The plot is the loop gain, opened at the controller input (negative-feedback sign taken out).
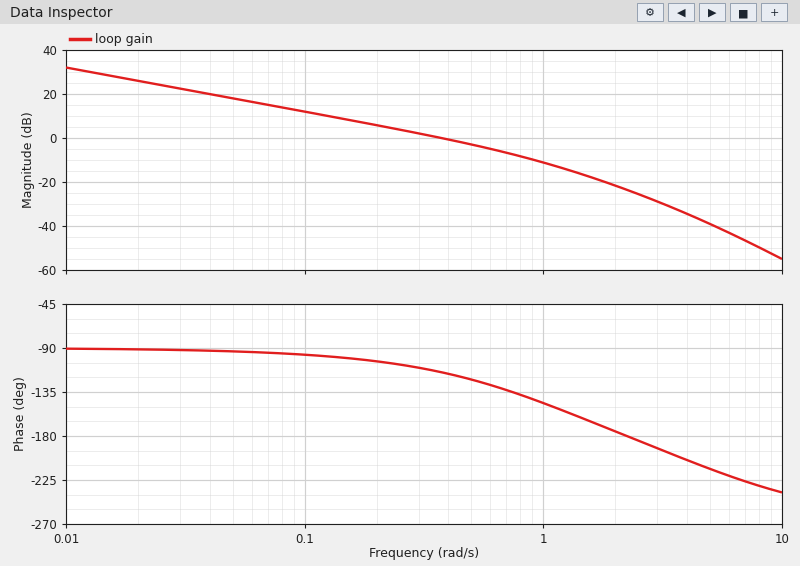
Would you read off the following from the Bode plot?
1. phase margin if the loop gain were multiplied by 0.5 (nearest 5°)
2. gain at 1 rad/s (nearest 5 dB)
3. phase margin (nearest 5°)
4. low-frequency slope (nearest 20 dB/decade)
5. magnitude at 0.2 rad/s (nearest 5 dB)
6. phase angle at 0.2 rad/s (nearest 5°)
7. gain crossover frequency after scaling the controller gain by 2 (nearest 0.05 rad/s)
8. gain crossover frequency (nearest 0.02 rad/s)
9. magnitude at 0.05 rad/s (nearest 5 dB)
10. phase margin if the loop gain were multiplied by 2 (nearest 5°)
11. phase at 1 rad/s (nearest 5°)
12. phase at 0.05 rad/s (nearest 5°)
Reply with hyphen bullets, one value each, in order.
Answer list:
- 75°
- -10 dB
- 65°
- -20 dB/decade
- 5 dB
- -105°
- 0.65 rad/s
- 0.38 rad/s
- 20 dB
- 50°
- -145°
- -95°
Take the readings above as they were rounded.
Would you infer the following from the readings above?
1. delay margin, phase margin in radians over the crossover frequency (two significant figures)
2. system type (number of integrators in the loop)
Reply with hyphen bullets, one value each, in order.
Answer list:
- 3.0 s
- 1
